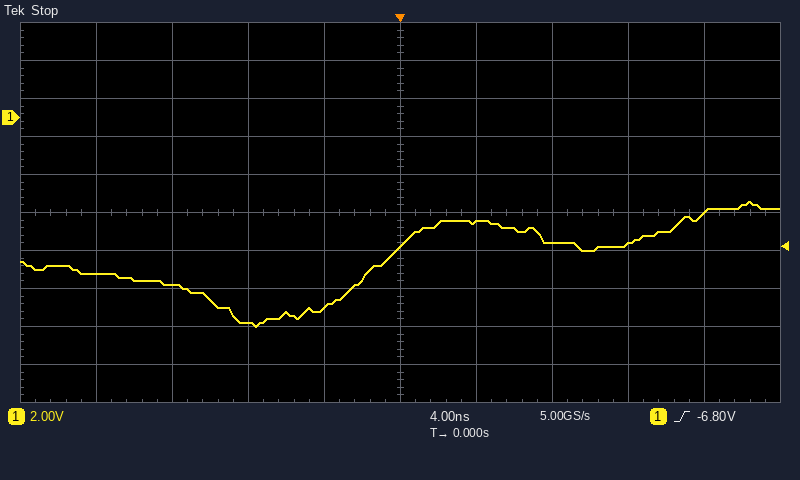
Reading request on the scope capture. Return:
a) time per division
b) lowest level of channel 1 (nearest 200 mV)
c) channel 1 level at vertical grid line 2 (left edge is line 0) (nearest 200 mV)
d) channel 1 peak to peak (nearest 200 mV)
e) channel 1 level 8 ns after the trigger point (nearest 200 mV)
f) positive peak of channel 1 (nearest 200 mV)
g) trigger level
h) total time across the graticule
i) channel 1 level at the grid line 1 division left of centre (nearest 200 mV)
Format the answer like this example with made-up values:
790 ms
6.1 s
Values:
4 ns
-11.0 V
-8.8 V
6.6 V
-6.6 V
-4.4 V
-6.80 V
40 ns
-10.0 V
